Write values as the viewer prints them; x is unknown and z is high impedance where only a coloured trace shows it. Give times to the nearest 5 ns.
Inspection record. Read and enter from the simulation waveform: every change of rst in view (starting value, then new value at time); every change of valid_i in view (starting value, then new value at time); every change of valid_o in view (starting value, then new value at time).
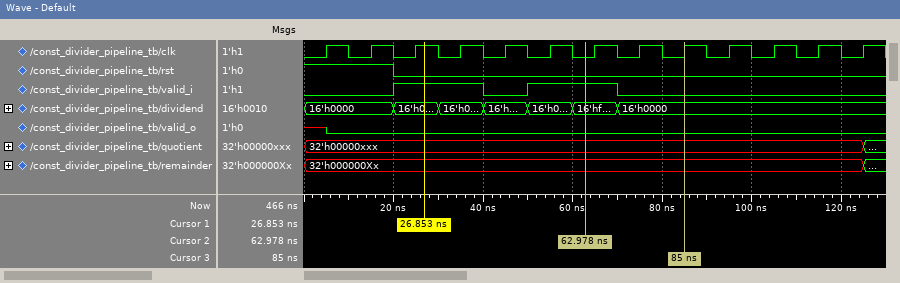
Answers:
1, 0 at 20 ns
0, 1 at 20 ns, 0 at 40 ns, 1 at 50 ns, 0 at 70 ns
x, 0 at 5 ns
